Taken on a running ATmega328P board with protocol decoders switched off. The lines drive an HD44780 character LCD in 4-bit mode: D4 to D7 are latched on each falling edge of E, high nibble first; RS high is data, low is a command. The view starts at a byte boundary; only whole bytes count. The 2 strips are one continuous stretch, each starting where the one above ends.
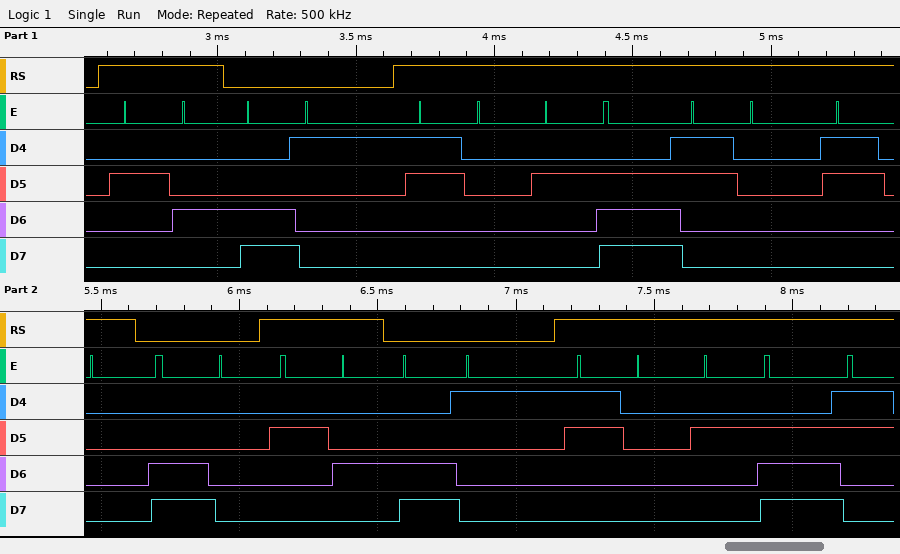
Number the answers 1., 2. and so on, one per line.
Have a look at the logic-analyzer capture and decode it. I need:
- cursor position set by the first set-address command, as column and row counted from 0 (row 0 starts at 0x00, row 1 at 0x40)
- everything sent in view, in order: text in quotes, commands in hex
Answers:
1. column 1, row 1
2. "$" 0xC1 "0.00" 0xC0 "$" 0xC1 "0."
